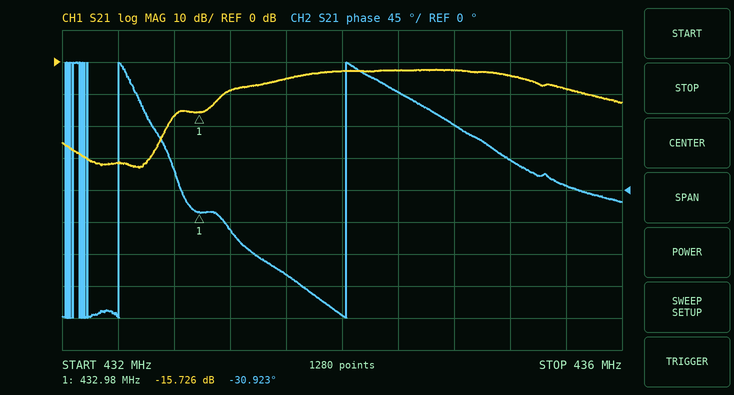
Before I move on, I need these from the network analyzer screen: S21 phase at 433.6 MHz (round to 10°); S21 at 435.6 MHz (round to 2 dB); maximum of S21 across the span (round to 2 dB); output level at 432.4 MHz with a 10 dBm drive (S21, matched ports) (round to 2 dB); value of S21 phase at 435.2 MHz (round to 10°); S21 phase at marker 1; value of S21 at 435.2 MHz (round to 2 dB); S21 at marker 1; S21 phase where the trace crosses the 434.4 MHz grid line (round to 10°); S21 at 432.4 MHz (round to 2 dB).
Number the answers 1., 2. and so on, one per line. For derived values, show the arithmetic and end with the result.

1. -120°
2. -8 dB
3. -2 dB
4. 10 dBm + (-32 dB) = -22 dBm
5. 40°
6. -30.923°
7. -4 dB
8. -15.726 dB
9. 140°
10. -32 dB
